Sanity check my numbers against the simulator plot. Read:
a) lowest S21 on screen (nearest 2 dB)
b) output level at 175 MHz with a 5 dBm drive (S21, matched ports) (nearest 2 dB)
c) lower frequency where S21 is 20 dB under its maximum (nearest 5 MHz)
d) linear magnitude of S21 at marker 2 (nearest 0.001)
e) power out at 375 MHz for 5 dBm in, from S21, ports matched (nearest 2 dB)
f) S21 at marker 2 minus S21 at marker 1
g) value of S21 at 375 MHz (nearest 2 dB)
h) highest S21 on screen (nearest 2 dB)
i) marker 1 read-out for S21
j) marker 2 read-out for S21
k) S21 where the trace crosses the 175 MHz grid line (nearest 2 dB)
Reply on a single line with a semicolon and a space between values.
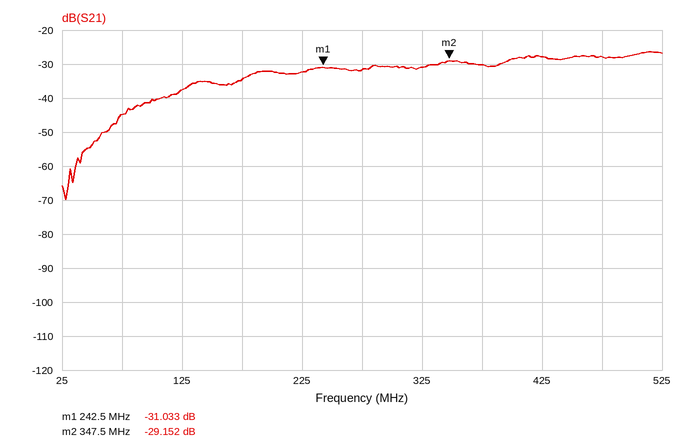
-70 dB; -30 dBm; 70 MHz; 0.035; -26 dBm; 1.881 dB; -30 dB; -26 dB; -31.033 dB; -29.152 dB; -34 dB
